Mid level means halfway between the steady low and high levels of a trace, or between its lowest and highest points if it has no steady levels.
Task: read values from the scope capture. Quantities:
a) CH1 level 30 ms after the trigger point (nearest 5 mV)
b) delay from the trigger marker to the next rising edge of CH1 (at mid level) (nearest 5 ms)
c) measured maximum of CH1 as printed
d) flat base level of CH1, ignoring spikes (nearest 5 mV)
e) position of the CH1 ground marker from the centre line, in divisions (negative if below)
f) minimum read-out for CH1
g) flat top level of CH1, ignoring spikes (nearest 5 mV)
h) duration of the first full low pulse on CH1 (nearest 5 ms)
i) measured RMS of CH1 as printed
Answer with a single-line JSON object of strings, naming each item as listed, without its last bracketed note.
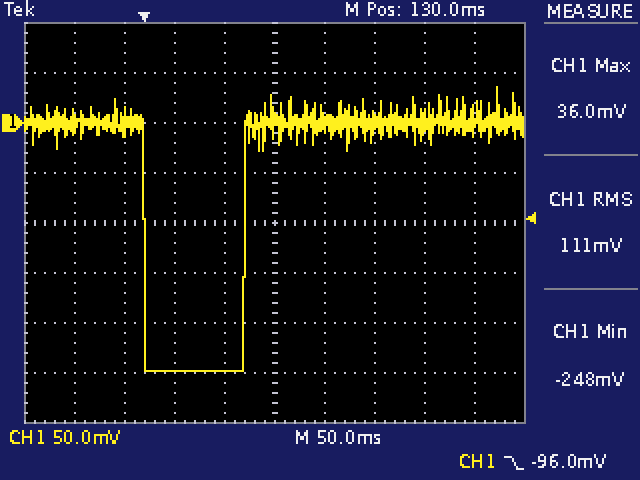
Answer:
{"CH1 level 30 ms after the trigger point": "-250 mV", "delay from the trigger marker to the next rising edge of CH1 (at mid level)": "100 ms", "measured maximum of CH1 as printed": "36.0 mV", "flat base level of CH1, ignoring spikes": "-250 mV", "position of the CH1 ground marker from the centre line, in divisions": "+2.0 div", "minimum read-out for CH1": "-248 mV", "flat top level of CH1, ignoring spikes": "0 mV", "duration of the first full low pulse on CH1": "100 ms", "measured RMS of CH1 as printed": "111 mV"}
